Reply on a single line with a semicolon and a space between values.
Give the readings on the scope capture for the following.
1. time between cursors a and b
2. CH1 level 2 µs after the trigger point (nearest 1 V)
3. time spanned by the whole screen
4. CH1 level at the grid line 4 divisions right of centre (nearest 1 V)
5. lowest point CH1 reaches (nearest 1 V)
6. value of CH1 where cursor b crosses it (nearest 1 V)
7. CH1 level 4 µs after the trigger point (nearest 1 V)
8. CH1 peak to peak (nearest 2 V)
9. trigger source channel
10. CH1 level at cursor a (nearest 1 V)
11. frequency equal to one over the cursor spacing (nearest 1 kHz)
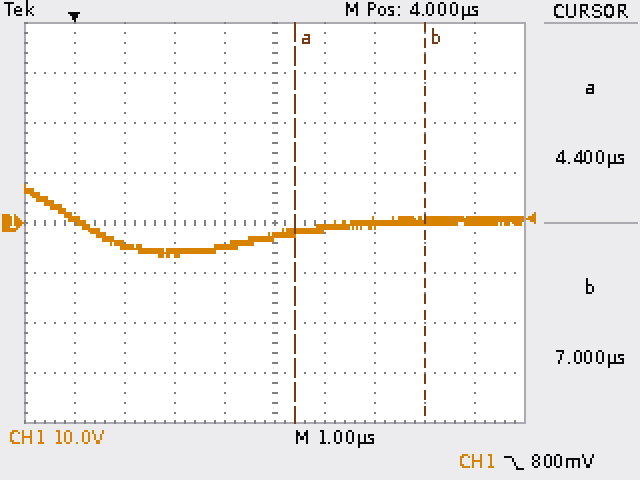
2.6 µs; -6 V; 10 µs; 0 V; -7 V; 0 V; -3 V; 14 V; CH1; -2 V; 385 kHz
